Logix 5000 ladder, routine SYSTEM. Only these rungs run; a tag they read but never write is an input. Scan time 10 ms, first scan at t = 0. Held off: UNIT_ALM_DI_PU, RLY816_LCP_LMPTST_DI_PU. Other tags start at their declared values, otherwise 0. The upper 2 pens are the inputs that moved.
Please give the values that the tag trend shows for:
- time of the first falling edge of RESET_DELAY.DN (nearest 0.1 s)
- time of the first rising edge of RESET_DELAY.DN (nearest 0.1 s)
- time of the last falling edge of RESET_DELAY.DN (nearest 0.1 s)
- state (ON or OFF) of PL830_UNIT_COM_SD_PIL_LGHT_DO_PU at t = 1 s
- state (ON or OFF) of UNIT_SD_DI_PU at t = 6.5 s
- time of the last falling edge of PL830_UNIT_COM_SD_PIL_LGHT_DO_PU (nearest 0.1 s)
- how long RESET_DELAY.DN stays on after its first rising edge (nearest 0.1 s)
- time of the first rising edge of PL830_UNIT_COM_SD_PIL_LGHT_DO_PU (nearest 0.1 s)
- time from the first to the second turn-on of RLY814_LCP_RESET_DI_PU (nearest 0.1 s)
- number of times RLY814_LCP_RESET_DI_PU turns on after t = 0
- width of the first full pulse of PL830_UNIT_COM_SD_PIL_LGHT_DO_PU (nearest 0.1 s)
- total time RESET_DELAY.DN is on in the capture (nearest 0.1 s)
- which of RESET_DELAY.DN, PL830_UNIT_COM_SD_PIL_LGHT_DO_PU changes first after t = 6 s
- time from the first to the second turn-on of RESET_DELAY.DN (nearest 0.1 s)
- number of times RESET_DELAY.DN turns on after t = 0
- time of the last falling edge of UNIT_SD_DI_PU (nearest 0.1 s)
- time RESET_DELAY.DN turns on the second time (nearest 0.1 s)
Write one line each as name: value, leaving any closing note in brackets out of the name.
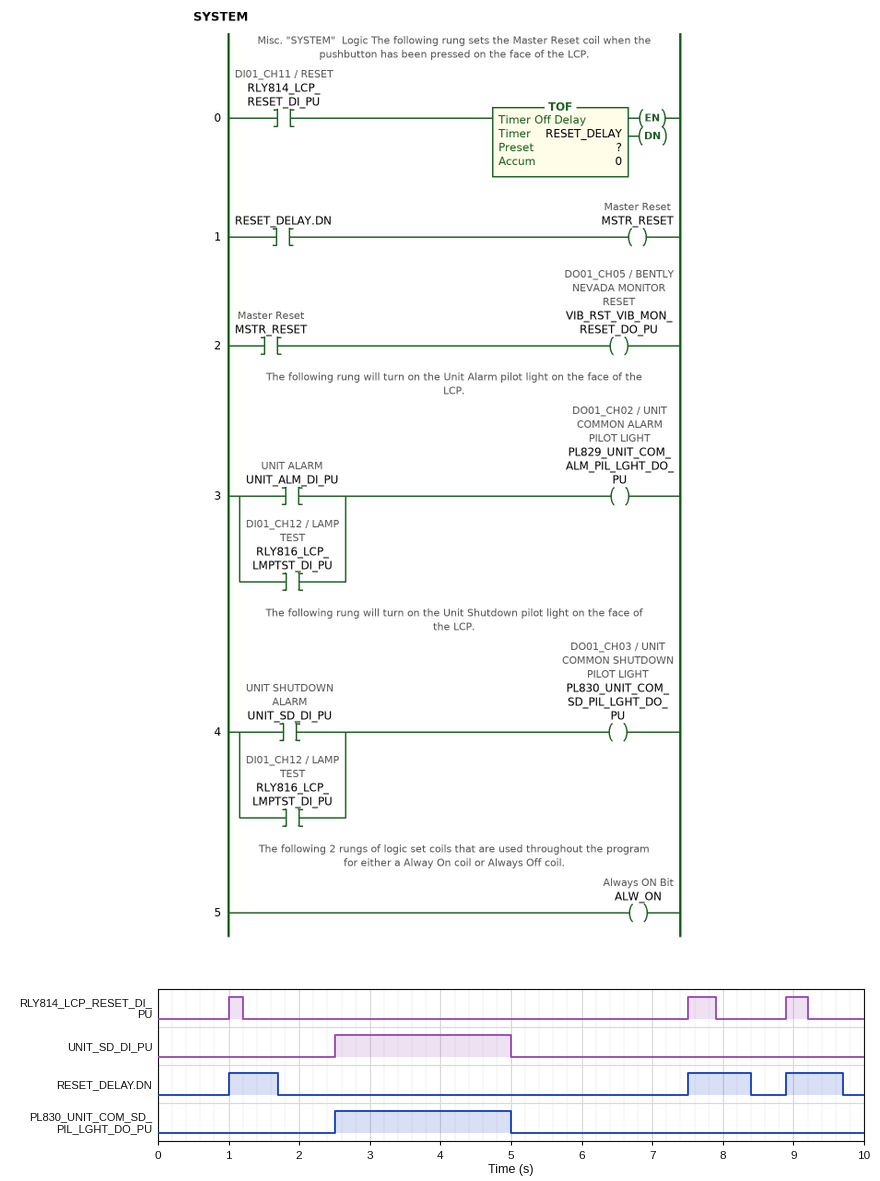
time of the first falling edge of RESET_DELAY.DN: 1.7 s
time of the first rising edge of RESET_DELAY.DN: 1.0 s
time of the last falling edge of RESET_DELAY.DN: 9.7 s
state (ON or OFF) of PL830_UNIT_COM_SD_PIL_LGHT_DO_PU at t = 1 s: OFF
state (ON or OFF) of UNIT_SD_DI_PU at t = 6.5 s: OFF
time of the last falling edge of PL830_UNIT_COM_SD_PIL_LGHT_DO_PU: 5.0 s
how long RESET_DELAY.DN stays on after its first rising edge: 0.7 s
time of the first rising edge of PL830_UNIT_COM_SD_PIL_LGHT_DO_PU: 2.5 s
time from the first to the second turn-on of RLY814_LCP_RESET_DI_PU: 6.5 s
number of times RLY814_LCP_RESET_DI_PU turns on after t = 0: 3
width of the first full pulse of PL830_UNIT_COM_SD_PIL_LGHT_DO_PU: 2.5 s
total time RESET_DELAY.DN is on in the capture: 2.4 s
which of RESET_DELAY.DN, PL830_UNIT_COM_SD_PIL_LGHT_DO_PU changes first after t = 6 s: RESET_DELAY.DN
time from the first to the second turn-on of RESET_DELAY.DN: 6.5 s
number of times RESET_DELAY.DN turns on after t = 0: 3
time of the last falling edge of UNIT_SD_DI_PU: 5.0 s
time RESET_DELAY.DN turns on the second time: 7.5 s
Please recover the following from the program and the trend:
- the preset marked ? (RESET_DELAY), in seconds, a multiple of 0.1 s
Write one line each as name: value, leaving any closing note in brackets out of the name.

the preset marked ? (RESET_DELAY), in seconds, a multiple of 0.1 s: 0.5 s
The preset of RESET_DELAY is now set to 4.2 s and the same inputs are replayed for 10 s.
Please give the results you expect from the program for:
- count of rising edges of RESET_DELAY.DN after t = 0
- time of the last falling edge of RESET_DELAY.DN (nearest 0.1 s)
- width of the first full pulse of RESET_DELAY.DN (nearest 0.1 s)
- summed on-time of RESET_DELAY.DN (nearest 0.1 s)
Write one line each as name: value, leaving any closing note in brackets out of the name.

count of rising edges of RESET_DELAY.DN after t = 0: 2
time of the last falling edge of RESET_DELAY.DN: 5.4 s
width of the first full pulse of RESET_DELAY.DN: 4.4 s
summed on-time of RESET_DELAY.DN: 6.9 s
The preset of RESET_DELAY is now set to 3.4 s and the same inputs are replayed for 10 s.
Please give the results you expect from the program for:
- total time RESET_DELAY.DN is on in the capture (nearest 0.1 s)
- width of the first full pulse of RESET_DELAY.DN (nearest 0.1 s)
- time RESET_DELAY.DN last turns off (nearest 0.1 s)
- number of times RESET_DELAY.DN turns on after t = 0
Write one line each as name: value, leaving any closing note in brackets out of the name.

total time RESET_DELAY.DN is on in the capture: 6.1 s
width of the first full pulse of RESET_DELAY.DN: 3.6 s
time RESET_DELAY.DN last turns off: 4.6 s
number of times RESET_DELAY.DN turns on after t = 0: 2
